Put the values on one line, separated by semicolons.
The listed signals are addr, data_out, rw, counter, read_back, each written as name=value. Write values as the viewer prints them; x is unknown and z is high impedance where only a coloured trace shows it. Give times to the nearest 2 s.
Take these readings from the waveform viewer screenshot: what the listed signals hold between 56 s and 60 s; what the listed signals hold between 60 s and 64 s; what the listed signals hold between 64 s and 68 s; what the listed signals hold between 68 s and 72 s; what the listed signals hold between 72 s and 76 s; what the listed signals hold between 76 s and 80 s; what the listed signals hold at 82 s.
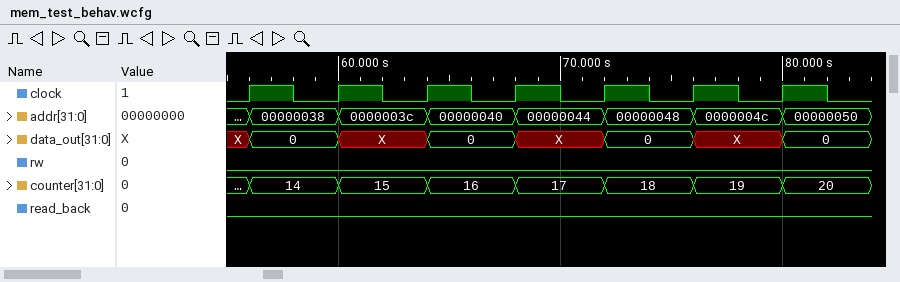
addr=00000038, data_out=0, rw=0, counter=14, read_back=0; addr=0000003c, data_out=X, rw=0, counter=15, read_back=0; addr=00000040, data_out=0, rw=0, counter=16, read_back=0; addr=00000044, data_out=X, rw=0, counter=17, read_back=0; addr=00000048, data_out=0, rw=0, counter=18, read_back=0; addr=0000004c, data_out=X, rw=0, counter=19, read_back=0; addr=00000050, data_out=0, rw=0, counter=20, read_back=0
